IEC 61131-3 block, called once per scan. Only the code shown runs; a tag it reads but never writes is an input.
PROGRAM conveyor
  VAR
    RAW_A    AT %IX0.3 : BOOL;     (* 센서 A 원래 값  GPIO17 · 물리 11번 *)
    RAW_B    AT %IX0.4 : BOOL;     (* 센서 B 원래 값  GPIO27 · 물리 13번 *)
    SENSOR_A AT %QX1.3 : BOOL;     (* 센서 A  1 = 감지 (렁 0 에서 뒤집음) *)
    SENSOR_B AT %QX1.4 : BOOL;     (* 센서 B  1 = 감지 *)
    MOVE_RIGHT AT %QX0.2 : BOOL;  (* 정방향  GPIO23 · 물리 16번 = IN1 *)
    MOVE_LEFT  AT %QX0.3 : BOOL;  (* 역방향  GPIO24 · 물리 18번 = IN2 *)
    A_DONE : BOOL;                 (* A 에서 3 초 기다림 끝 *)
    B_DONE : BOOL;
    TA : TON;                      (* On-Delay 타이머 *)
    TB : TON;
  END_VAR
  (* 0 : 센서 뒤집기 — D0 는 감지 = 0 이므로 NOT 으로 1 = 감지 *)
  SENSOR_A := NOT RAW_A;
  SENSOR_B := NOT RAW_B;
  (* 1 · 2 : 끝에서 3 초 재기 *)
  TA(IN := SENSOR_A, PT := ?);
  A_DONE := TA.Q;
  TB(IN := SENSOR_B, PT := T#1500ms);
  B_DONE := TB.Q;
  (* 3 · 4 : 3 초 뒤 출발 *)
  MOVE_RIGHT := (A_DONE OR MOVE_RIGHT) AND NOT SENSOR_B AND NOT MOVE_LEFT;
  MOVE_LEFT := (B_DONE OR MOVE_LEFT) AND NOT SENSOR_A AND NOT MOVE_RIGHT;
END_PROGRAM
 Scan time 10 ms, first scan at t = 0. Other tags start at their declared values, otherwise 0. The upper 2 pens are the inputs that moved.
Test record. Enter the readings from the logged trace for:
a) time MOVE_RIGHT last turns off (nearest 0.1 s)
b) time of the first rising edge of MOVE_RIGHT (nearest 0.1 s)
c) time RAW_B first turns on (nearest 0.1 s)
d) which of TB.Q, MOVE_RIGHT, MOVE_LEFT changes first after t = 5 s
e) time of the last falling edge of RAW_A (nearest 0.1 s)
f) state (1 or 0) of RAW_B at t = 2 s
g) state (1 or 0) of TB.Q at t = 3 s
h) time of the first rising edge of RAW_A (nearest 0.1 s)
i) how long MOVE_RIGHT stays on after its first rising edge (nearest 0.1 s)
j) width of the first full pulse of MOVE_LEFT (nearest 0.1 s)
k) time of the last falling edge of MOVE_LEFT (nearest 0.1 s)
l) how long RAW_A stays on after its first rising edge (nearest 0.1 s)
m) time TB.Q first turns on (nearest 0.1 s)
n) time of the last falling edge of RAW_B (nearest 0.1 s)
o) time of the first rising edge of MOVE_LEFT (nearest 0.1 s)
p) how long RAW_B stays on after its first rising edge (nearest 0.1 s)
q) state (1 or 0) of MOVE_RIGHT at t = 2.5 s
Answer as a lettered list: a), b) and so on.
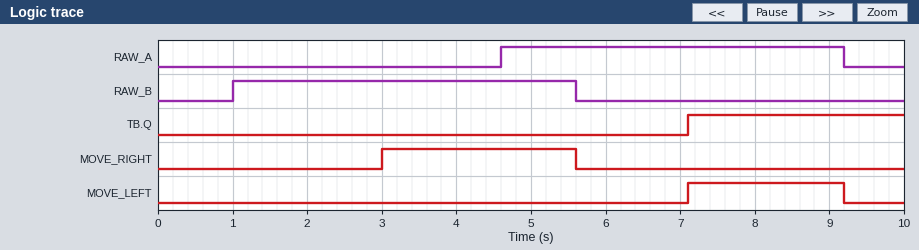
a) 5.6 s
b) 3.0 s
c) 1.0 s
d) MOVE_RIGHT
e) 9.2 s
f) 1
g) 0
h) 4.6 s
i) 2.6 s
j) 2.1 s
k) 9.2 s
l) 4.6 s
m) 7.1 s
n) 5.6 s
o) 7.1 s
p) 4.6 s
q) 0
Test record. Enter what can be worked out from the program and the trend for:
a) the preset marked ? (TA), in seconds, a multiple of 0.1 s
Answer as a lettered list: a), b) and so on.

a) 3.0 s
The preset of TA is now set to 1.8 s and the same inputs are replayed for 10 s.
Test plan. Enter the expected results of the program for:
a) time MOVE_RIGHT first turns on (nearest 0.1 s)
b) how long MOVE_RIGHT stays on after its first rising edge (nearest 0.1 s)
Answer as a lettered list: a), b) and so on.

a) 1.8 s
b) 3.8 s
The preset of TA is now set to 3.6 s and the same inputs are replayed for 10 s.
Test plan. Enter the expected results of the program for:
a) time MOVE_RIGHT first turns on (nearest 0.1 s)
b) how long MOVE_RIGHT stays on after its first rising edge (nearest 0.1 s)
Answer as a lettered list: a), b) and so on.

a) 3.6 s
b) 2.0 s
